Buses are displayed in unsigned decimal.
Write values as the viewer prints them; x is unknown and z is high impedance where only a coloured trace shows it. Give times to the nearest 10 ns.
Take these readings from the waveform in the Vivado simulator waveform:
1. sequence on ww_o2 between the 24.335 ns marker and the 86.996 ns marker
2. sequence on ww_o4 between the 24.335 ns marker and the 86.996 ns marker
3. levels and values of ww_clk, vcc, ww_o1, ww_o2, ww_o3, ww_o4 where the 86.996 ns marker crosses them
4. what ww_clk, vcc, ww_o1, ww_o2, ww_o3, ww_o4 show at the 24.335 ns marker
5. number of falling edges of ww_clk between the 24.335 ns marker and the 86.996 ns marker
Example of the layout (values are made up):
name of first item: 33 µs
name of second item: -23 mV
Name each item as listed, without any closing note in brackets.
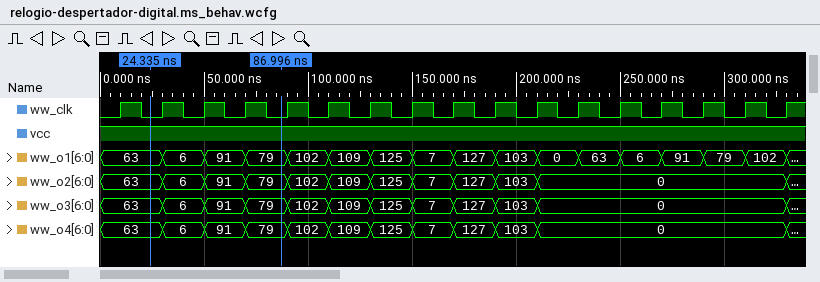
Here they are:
sequence on ww_o2 between the 24.335 ns marker and the 86.996 ns marker: 63, 6, 91, 79
sequence on ww_o4 between the 24.335 ns marker and the 86.996 ns marker: 63, 6, 91, 79
levels and values of ww_clk, vcc, ww_o1, ww_o2, ww_o3, ww_o4 where the 86.996 ns marker crosses them: ww_clk=0, vcc=1, ww_o1=79, ww_o2=79, ww_o3=79, ww_o4=79
what ww_clk, vcc, ww_o1, ww_o2, ww_o3, ww_o4 show at the 24.335 ns marker: ww_clk=0, vcc=1, ww_o1=63, ww_o2=63, ww_o3=63, ww_o4=63
number of falling edges of ww_clk between the 24.335 ns marker and the 86.996 ns marker: 3
